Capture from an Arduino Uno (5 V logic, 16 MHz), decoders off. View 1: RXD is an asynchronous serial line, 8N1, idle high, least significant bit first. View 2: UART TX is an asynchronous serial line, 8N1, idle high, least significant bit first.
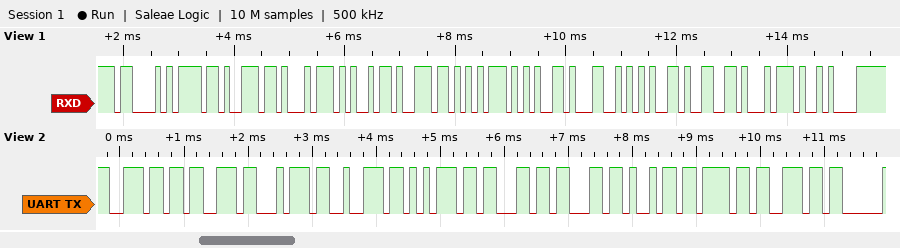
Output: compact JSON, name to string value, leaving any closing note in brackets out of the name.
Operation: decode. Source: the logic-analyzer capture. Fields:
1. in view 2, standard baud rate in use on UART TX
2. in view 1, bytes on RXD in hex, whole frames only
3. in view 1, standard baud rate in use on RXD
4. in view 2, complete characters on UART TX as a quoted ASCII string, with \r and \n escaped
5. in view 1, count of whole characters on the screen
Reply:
{"in view 2, standard baud rate in use on UART TX": "9600 baud", "in view 1, bytes on RXD in hex, whole frames only": "43 6F 6E 74 69 6E 75 65 4C 65 66 74 0A", "in view 1, standard baud rate in use on RXD": "9600 baud", "in view 2, complete characters on UART TX as a quoted ASCII string, with \\r and \\n escaped": "\"nstruccion\"", "in view 1, count of whole characters on the screen": "13"}
